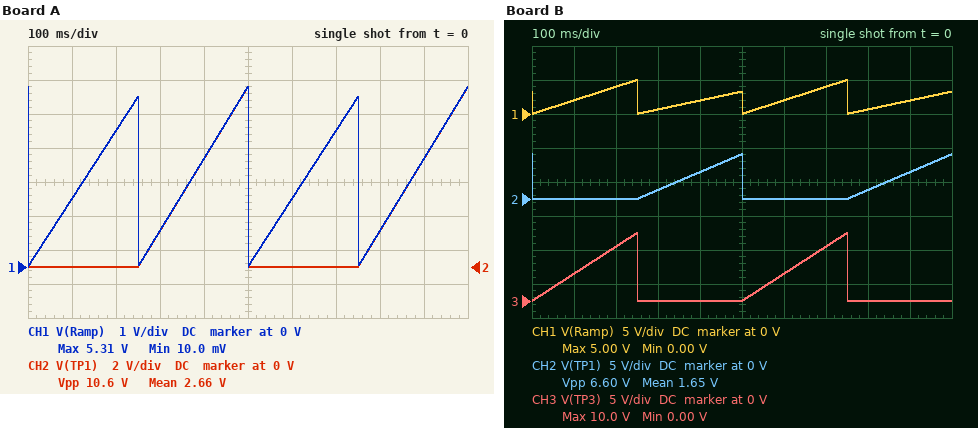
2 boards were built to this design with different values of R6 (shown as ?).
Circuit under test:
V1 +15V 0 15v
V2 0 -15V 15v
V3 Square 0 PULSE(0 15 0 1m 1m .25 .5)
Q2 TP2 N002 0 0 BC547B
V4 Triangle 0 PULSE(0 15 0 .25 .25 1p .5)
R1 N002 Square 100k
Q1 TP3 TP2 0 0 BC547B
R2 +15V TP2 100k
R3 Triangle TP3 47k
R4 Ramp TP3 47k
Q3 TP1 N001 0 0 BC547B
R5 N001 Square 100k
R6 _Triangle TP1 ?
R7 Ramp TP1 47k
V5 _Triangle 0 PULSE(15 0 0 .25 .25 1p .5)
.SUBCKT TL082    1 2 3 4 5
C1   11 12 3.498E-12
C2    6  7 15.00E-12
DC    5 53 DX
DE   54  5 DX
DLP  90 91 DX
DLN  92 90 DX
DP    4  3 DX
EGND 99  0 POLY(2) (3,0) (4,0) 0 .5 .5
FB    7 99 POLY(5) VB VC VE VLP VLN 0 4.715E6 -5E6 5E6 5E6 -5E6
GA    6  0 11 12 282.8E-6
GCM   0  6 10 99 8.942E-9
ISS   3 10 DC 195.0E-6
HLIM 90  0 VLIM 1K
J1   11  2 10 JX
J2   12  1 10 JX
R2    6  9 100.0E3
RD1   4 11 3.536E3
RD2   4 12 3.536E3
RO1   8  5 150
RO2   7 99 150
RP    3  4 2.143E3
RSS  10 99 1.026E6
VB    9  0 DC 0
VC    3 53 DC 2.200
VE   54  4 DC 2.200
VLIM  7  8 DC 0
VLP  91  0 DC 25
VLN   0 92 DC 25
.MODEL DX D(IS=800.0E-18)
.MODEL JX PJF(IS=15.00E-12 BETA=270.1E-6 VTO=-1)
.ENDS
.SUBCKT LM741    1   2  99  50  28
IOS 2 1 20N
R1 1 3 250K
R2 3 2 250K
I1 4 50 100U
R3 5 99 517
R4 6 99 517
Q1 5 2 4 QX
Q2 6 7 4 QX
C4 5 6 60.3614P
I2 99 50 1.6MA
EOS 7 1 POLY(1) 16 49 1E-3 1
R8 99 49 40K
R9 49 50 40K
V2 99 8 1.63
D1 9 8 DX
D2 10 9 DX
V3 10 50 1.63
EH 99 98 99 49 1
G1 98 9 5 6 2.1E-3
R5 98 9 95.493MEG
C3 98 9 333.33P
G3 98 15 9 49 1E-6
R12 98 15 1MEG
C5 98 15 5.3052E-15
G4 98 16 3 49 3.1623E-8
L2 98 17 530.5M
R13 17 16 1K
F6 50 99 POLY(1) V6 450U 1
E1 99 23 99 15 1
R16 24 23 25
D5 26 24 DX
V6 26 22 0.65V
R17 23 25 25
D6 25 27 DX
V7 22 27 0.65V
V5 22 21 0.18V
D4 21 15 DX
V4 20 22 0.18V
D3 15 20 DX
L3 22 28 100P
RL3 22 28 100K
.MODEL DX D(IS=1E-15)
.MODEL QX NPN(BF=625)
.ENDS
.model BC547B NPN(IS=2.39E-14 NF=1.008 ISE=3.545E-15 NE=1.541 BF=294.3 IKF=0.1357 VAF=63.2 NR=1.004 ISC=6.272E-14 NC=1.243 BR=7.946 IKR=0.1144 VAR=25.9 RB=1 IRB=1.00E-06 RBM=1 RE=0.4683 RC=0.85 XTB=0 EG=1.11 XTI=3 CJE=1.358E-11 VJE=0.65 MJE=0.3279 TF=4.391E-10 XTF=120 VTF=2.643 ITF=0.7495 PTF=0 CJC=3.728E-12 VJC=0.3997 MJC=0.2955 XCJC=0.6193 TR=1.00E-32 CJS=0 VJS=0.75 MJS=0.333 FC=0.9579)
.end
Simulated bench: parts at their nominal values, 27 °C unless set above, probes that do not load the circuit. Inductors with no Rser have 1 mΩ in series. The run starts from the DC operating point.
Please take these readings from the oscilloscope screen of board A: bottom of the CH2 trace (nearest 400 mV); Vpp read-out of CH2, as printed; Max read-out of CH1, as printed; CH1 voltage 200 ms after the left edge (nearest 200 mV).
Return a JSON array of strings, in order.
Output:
["0 V", "10.6 V", "5.31 V", "4.0 V"]
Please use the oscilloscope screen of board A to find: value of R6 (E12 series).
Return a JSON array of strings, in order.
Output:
["39 kΩ"]
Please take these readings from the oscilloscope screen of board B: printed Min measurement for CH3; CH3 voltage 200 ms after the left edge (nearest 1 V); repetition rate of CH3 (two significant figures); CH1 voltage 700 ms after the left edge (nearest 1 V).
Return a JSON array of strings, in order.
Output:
["0.00 V", "8 V", "2.0 Hz", "4 V"]
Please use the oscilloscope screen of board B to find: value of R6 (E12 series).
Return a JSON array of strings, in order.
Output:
["120 kΩ"]
